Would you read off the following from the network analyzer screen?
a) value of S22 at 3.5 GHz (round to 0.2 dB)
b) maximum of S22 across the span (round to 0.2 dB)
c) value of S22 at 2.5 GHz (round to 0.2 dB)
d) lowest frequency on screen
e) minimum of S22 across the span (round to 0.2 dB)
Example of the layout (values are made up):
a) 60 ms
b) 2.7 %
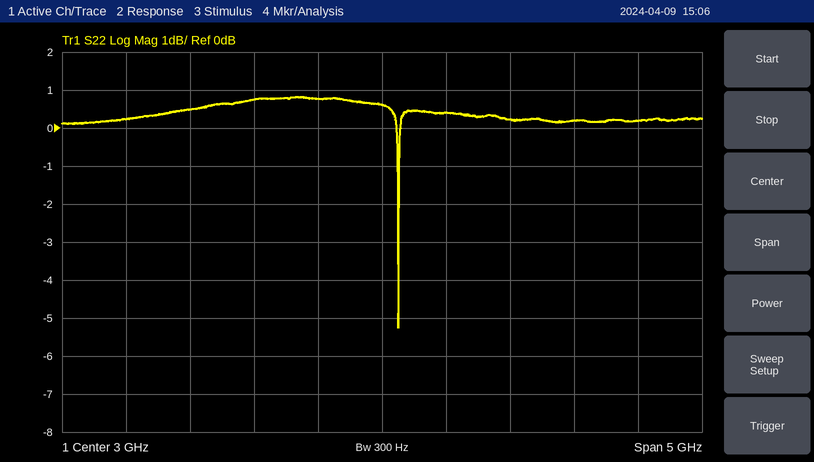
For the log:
a) 0.4 dB
b) 0.8 dB
c) 0.8 dB
d) 500 MHz
e) -5.2 dB
